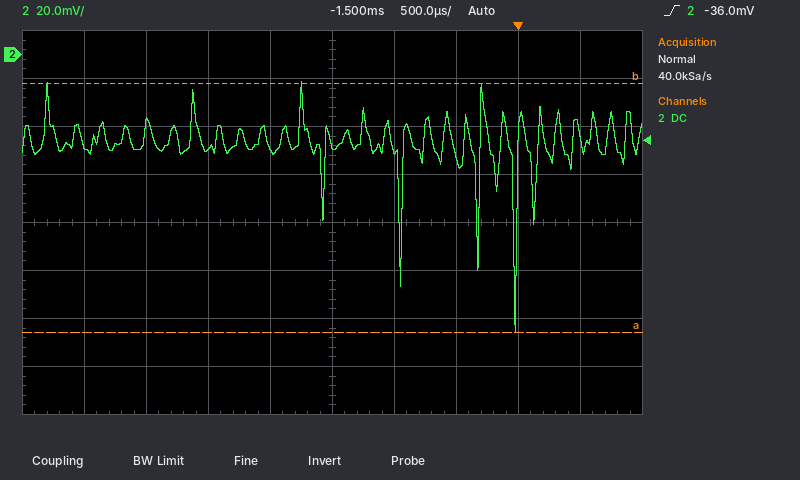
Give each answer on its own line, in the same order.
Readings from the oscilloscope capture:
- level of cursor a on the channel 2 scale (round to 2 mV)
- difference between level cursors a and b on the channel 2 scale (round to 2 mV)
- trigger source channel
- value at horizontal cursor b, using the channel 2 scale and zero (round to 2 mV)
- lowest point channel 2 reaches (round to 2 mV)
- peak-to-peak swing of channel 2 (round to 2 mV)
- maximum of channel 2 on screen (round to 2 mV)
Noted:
-116 mV
104 mV
channel 2
-12 mV
-116 mV
104 mV
-12 mV
